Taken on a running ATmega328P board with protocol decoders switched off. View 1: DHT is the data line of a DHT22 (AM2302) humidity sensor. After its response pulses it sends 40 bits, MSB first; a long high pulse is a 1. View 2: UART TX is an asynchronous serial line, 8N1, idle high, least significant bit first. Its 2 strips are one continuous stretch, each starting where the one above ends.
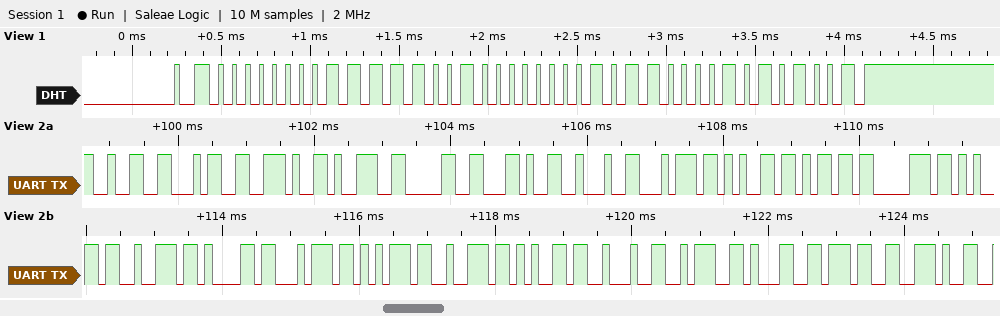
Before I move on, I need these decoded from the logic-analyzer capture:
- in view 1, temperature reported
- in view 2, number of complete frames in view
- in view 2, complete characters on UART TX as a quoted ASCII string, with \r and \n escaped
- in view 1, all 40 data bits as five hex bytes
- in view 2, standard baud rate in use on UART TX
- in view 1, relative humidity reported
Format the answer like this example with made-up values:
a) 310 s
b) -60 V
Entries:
a) 17.6 °C
b) 23
c) "24.90,\"temperature\":17."
d) 00 F9 00 B0 A9
e) 9600 baud
f) 24.9 %
